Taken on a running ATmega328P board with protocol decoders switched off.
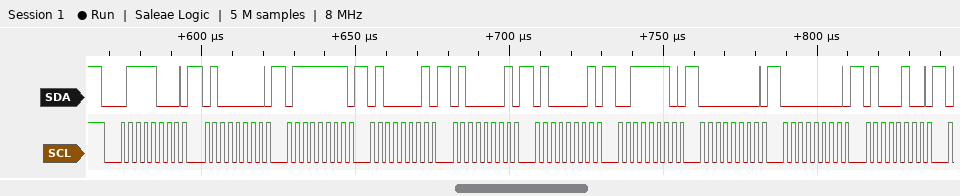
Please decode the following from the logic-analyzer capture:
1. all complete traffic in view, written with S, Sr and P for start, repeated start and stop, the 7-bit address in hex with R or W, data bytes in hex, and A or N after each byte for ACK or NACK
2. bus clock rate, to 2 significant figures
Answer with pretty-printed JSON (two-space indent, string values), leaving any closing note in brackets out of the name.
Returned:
{
  "all complete traffic in view, written with S, Sr and P for start, repeated start and stop, the 7-bit address in hex with R or W, data bytes in hex, and A or N after each byte for ACK or NACK": "S 3CW A 40 A 7F A 41 A 41 A 41 A 3E A 00 A 00 A 44 A",
  "bus clock rate, to 2 significant figures": "400 kHz"
}
